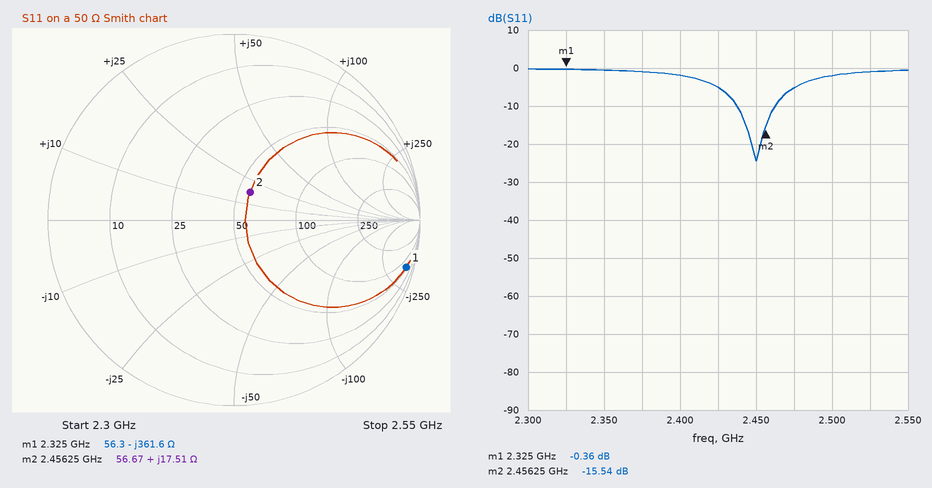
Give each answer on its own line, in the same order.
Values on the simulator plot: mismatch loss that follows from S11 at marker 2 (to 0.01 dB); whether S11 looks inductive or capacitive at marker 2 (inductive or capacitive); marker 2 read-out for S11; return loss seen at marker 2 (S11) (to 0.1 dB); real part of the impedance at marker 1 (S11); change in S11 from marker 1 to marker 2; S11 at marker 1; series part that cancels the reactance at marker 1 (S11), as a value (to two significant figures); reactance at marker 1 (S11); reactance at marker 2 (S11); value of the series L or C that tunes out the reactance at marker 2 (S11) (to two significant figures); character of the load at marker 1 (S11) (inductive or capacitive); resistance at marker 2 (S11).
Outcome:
0.12 dB
inductive
-15.54 dB
15.2 dB
56.3 Ω
-15.18 dB
-0.36 dB
25 nH
-361.6 Ω
+17.51 Ω
3.7 pF
capacitive
56.67 Ω
